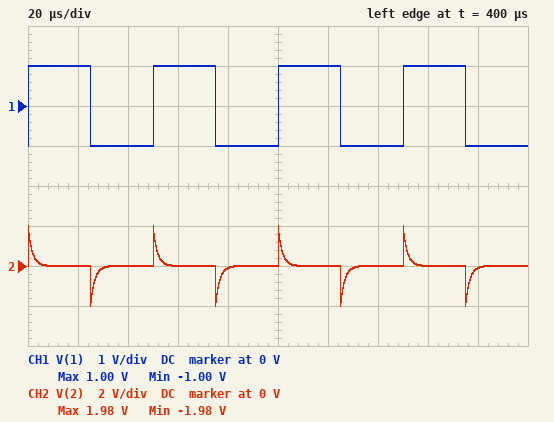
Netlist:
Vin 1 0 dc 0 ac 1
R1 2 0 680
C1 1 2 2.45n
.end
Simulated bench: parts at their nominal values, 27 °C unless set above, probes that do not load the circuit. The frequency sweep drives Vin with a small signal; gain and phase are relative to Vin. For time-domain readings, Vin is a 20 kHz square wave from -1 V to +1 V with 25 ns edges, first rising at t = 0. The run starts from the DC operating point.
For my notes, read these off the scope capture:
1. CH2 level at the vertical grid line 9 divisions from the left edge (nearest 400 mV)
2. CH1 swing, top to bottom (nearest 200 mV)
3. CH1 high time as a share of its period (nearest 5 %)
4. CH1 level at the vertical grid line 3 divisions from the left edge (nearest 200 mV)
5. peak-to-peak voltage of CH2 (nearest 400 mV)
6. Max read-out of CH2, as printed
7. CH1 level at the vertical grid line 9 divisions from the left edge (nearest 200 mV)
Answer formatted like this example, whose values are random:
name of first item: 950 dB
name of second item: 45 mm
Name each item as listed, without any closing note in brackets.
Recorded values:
CH2 level at the vertical grid line 9 divisions from the left edge: 0 V
CH1 swing, top to bottom: 2.0 V
CH1 high time as a share of its period: 50 %
CH1 level at the vertical grid line 3 divisions from the left edge: 1.0 V
peak-to-peak voltage of CH2: 4.0 V
Max read-out of CH2, as printed: 1.98 V
CH1 level at the vertical grid line 9 divisions from the left edge: -1.0 V
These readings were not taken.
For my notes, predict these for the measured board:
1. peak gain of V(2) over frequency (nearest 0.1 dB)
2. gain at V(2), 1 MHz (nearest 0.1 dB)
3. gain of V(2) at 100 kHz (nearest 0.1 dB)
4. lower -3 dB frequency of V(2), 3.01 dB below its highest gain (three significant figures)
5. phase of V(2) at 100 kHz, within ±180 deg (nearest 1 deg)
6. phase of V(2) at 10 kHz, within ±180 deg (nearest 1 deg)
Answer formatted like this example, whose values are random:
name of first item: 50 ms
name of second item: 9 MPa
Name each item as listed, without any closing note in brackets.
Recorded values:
peak gain of V(2) over frequency: 0 dB
gain at V(2), 1 MHz: 0 dB
gain of V(2) at 100 kHz: -2.8 dB
lower -3 dB frequency of V(2), 3.01 dB below its highest gain: 95.5 kHz
phase of V(2) at 100 kHz, within ±180 deg: 44 deg
phase of V(2) at 10 kHz, within ±180 deg: 84 deg
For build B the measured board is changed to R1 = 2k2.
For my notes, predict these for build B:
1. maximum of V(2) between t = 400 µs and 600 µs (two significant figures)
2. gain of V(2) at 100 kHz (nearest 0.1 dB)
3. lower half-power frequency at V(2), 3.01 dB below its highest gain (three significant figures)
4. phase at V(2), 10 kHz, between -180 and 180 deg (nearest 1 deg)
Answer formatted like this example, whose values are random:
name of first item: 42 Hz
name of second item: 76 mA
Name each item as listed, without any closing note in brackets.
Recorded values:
maximum of V(2) between t = 400 µs and 600 µs: 2.0 V
gain of V(2) at 100 kHz: -0.4 dB
lower half-power frequency at V(2), 3.01 dB below its highest gain: 29.5 kHz
phase at V(2), 10 kHz, between -180 and 180 deg: 71 deg
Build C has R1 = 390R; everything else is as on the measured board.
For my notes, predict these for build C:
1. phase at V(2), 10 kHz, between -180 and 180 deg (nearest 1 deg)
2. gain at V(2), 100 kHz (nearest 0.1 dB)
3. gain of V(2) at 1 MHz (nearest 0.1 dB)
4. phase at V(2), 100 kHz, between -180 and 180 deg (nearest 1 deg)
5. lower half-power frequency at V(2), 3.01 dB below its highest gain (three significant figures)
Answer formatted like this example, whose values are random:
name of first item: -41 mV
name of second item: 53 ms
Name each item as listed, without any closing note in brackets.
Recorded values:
phase at V(2), 10 kHz, between -180 and 180 deg: 87 deg
gain at V(2), 100 kHz: -5.8 dB
gain of V(2) at 1 MHz: -0.1 dB
phase at V(2), 100 kHz, between -180 and 180 deg: 59 deg
lower half-power frequency at V(2), 3.01 dB below its highest gain: 167 kHz
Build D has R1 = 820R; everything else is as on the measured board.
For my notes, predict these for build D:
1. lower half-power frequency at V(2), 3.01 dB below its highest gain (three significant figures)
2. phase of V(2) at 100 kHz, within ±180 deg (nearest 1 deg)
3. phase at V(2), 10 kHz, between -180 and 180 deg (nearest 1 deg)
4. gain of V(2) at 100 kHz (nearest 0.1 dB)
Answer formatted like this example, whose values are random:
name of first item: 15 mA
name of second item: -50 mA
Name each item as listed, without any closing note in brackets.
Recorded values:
lower half-power frequency at V(2), 3.01 dB below its highest gain: 79.2 kHz
phase of V(2) at 100 kHz, within ±180 deg: 38 deg
phase at V(2), 10 kHz, between -180 and 180 deg: 83 deg
gain of V(2) at 100 kHz: -2.1 dB
